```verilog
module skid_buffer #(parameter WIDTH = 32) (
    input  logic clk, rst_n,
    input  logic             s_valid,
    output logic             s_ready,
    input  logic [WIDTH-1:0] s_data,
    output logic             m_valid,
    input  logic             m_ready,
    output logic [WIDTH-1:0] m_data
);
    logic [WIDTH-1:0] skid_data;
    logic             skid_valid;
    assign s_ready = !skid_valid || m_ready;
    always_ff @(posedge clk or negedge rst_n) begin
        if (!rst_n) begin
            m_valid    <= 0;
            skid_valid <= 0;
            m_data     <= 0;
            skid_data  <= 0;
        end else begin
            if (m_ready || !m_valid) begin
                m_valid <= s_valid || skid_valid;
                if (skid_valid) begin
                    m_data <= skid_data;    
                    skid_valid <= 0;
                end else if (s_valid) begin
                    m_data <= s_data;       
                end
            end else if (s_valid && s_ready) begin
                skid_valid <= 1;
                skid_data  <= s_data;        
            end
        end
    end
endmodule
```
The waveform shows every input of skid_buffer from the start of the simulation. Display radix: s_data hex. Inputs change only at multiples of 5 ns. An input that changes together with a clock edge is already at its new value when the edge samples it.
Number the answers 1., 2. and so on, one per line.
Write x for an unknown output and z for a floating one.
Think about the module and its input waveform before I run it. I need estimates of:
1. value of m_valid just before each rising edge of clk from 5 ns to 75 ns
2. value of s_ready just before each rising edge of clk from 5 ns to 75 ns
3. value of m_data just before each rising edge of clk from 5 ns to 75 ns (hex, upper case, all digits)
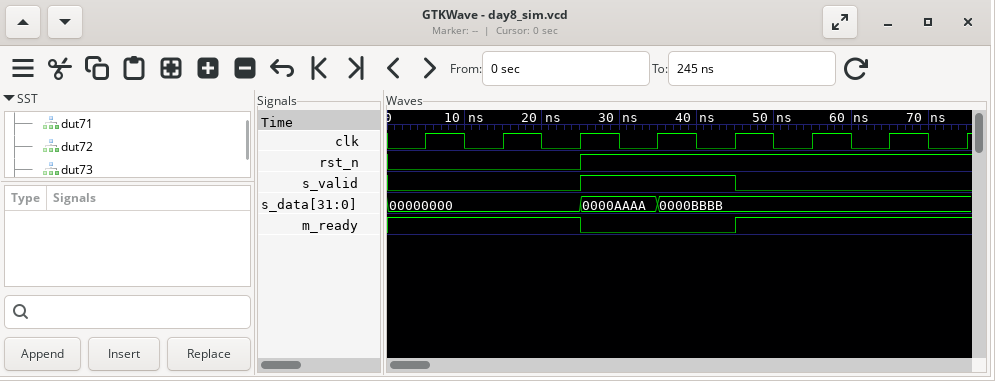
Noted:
1. 0 0 0 1 1 1 0 0
2. 1 1 1 1 0 1 1 1
3. 00000000, 00000000, 00000000, 0000AAAA, 0000AAAA, 0000BBBB, 0000BBBB, 0000BBBB
